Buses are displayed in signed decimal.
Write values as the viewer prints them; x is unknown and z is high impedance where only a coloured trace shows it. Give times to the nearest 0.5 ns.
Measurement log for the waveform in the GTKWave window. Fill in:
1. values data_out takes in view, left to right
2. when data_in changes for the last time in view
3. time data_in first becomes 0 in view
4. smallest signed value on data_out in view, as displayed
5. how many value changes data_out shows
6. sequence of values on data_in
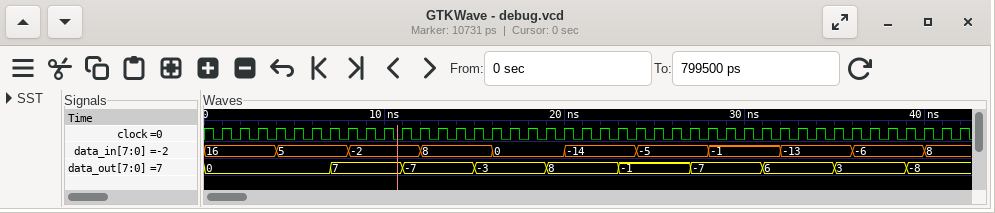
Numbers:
0, 7, -7, -3, 8, -1, -7, 6, 3, -8
40 ns
16 ns
-8
9
16, 5, -2, 8, 0, -14, -5, -1, -13, -6, 8
